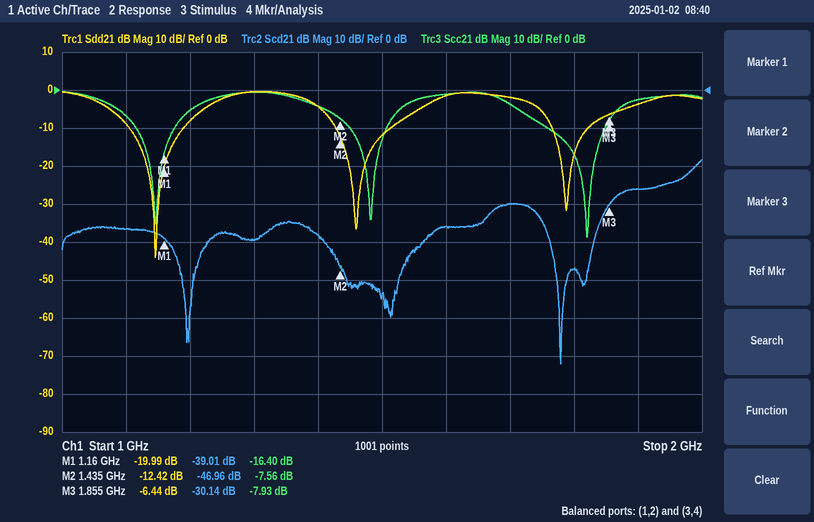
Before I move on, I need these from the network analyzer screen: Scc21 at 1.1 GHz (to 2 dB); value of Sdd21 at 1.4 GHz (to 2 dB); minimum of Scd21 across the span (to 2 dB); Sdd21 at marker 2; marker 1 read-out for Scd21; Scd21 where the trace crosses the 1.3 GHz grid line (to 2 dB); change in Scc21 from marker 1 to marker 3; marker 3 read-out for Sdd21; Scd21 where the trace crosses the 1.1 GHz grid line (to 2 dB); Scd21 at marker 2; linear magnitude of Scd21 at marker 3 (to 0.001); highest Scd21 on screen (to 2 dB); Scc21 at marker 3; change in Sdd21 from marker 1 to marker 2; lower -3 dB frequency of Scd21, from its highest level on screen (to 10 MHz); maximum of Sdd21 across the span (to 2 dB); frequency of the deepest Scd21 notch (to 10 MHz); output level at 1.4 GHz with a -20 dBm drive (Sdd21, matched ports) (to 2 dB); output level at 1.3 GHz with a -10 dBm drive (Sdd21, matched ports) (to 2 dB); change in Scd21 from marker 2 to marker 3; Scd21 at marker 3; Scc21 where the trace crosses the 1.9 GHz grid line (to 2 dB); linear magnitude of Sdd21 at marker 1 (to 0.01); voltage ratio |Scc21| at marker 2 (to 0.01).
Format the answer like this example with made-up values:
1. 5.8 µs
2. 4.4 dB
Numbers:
1. -6 dB
2. -4 dB
3. -72 dB
4. -12.42 dB
5. -39.01 dB
6. -40 dB
7. 8.47 dB
8. -6.44 dB
9. -36 dB
10. -46.96 dB
11. 0.031
12. -18 dB
13. -7.93 dB
14. 7.57 dB
15. 1.98 GHz
16. 0 dB
17. 1.78 GHz
18. -24 dBm
19. -10 dBm
20. 16.82 dB
21. -30.14 dB
22. -2 dB
23. 0.10
24. 0.42
